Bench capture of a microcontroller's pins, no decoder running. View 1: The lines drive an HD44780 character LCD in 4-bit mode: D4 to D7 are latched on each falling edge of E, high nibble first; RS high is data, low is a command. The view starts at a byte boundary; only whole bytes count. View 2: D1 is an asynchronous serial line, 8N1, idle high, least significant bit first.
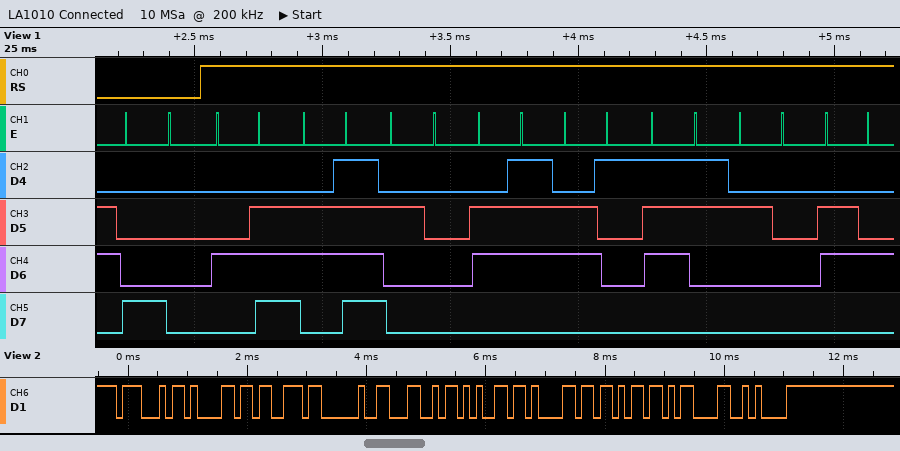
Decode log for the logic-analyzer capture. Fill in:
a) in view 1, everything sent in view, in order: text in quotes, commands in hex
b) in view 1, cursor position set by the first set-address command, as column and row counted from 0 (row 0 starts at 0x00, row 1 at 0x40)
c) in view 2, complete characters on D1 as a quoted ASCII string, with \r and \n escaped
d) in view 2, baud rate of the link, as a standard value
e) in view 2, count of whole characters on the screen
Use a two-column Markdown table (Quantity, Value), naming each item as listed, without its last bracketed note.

| Quantity | Value |
|---|---|
| in view 1, everything sent in view, in order: text in quotes, commands in hex | 0x80 "No gas d" |
| in view 1, cursor position set by the first set-address command, as column and row counted from 0 | column 0, row 0 |
| in view 2, complete characters on D1 as a quoted ASCII string, with \r and \n escaped | "Gas Leak\r\n" |
| in view 2, baud rate of the link, as a standard value | 9600 baud |
| in view 2, count of whole characters on the screen | 10 |
